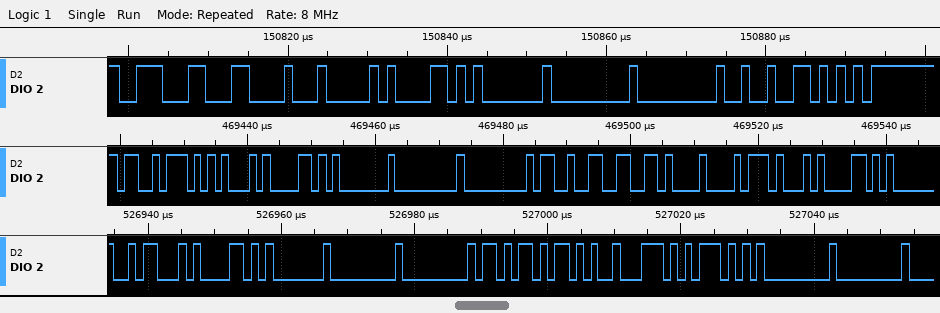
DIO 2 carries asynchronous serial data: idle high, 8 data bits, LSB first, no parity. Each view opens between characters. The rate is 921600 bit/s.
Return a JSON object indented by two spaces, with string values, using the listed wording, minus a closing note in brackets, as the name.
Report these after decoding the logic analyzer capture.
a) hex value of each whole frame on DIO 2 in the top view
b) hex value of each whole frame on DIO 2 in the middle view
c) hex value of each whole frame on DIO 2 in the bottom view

{
  "hex value of each whole frame on DIO 2 in the top view": "8E, 0C, 04, 61, 01, 00, 00, 92, D5",
  "hex value of each whole frame on DIO 2 in the middle view": "D3, 15, 61, 01, 00, 00, 93, 66, 08, 17, 61",
  "hex value of each whole frame on DIO 2 in the bottom view": "1A, 61, 01, 00, 00, 6B, 2B, 5C, 57, 00, 00"
}
